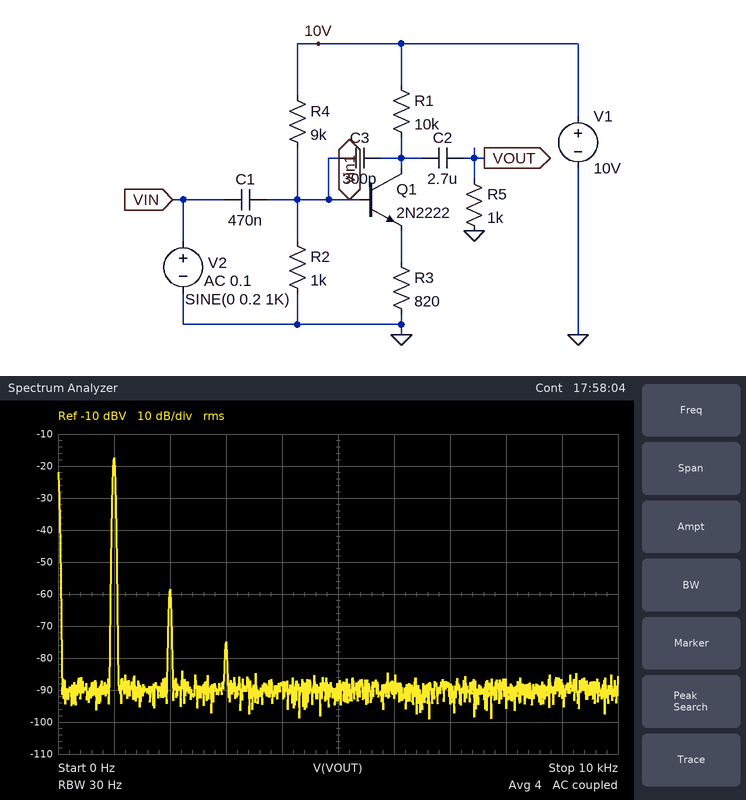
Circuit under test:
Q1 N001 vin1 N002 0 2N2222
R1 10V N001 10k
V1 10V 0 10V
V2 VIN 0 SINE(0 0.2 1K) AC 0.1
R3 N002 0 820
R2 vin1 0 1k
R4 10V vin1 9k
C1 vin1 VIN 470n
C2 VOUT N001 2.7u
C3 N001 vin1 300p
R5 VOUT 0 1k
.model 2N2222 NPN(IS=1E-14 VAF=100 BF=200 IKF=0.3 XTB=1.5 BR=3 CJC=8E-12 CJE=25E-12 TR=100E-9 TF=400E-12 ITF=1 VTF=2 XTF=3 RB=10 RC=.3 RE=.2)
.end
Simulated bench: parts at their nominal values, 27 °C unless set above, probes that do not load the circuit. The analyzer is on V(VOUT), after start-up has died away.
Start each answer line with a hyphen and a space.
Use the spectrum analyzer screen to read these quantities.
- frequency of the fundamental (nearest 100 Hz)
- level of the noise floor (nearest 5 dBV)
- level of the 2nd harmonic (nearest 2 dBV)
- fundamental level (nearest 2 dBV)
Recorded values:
- 1.0 kHz
- -90 dBV
- -58 dBV
- -18 dBV
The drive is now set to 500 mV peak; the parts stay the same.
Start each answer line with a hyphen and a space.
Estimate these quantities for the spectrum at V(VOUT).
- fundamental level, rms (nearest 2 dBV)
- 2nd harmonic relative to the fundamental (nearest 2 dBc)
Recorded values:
- -10 dBV
- -26 dBc
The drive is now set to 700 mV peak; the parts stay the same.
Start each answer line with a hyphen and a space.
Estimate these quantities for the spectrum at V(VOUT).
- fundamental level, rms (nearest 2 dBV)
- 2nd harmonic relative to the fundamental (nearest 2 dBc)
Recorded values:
- -8 dBV
- -18 dBc
